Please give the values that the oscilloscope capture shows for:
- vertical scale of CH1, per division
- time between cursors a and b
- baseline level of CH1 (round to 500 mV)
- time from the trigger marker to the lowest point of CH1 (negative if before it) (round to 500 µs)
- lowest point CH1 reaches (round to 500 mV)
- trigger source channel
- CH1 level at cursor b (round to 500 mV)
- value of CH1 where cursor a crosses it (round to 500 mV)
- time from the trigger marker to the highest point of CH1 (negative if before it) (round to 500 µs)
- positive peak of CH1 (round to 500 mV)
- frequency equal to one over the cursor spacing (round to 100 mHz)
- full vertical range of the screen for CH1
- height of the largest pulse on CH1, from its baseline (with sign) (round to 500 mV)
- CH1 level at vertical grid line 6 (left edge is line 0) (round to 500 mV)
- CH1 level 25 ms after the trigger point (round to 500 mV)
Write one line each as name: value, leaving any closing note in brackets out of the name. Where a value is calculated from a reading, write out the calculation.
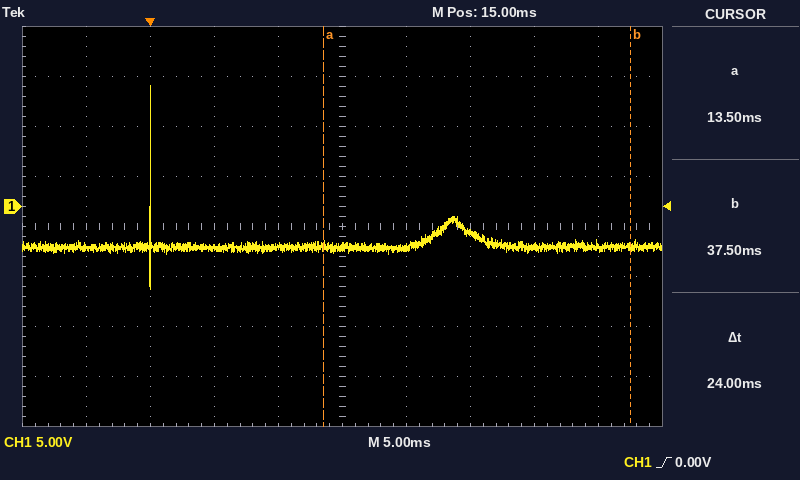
vertical scale of CH1, per division: 5 V
time between cursors a and b: 24 ms
baseline level of CH1: -4.0 V
time from the trigger marker to the lowest point of CH1 (negative if before it): 0.0 ms
lowest point CH1 reaches: -8.0 V
trigger source channel: CH1
CH1 level at cursor b: -4.0 V
value of CH1 where cursor a crosses it: -4.0 V
time from the trigger marker to the highest point of CH1 (negative if before it): 0.0 ms
positive peak of CH1: 12.0 V
frequency equal to one over the cursor spacing: 1 / 24 ms ≈ 41.7 Hz
full vertical range of the screen for CH1: 40 V
height of the largest pulse on CH1, from its baseline (with sign): 12.0 V − (-4.0 V) = +16.0 V
CH1 level at vertical grid line 6 (left edge is line 0): -4.0 V
CH1 level 25 ms after the trigger point: -2.5 V
